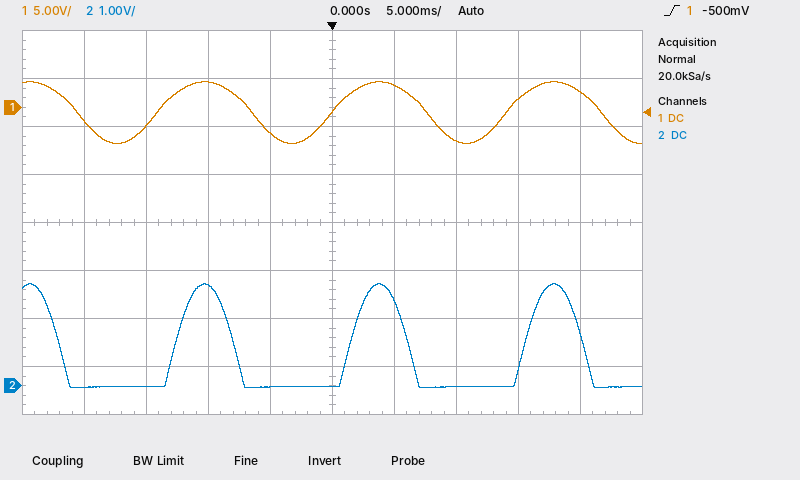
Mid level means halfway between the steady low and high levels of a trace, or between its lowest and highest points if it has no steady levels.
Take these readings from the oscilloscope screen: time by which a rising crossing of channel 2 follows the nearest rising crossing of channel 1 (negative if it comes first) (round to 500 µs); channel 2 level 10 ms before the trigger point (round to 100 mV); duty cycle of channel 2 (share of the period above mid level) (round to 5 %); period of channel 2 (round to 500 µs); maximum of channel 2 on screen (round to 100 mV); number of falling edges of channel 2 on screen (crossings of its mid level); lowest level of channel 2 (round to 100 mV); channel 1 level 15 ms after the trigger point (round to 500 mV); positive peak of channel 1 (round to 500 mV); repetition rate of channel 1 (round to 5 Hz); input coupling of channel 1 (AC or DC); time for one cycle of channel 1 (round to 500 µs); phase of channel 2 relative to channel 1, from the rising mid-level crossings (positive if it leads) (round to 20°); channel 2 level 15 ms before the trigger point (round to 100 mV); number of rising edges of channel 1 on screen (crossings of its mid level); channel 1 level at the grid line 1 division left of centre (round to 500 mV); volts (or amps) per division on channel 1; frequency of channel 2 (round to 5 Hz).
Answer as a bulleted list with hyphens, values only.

- +1.5 ms
- 2.1 V
- 30 %
- 14.0 ms
- 2.1 V
- 4
- 0.0 V
- 1.0 V
- 2.5 V
- 70 Hz
- DC
- 14.0 ms
- -40°
- 0.0 V
- 3
- -2.5 V
- 5 V
- 70 Hz
